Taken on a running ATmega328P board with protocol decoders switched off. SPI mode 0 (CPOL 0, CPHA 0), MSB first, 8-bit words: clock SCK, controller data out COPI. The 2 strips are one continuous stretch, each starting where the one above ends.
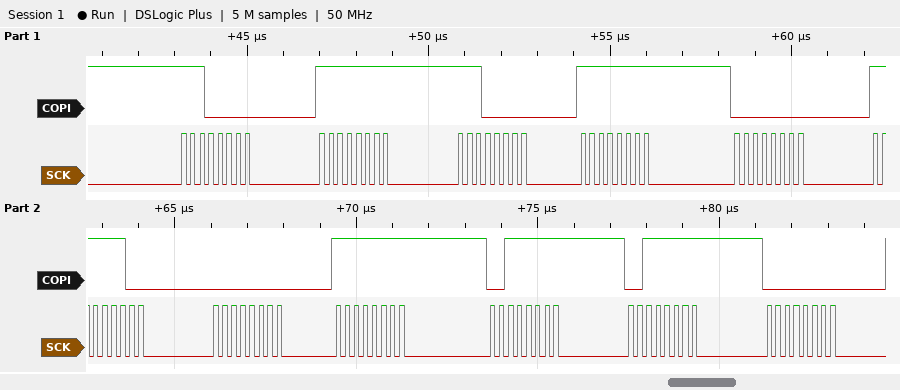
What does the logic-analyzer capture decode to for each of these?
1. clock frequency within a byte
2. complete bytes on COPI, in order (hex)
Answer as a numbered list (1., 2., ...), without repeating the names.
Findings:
1. 4 MHz
2. E0 FF E0 FF 00 FC 00 FF 3F 3F 00
